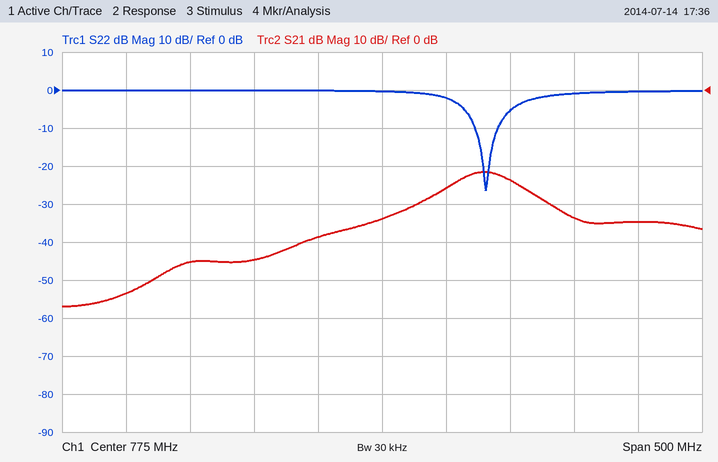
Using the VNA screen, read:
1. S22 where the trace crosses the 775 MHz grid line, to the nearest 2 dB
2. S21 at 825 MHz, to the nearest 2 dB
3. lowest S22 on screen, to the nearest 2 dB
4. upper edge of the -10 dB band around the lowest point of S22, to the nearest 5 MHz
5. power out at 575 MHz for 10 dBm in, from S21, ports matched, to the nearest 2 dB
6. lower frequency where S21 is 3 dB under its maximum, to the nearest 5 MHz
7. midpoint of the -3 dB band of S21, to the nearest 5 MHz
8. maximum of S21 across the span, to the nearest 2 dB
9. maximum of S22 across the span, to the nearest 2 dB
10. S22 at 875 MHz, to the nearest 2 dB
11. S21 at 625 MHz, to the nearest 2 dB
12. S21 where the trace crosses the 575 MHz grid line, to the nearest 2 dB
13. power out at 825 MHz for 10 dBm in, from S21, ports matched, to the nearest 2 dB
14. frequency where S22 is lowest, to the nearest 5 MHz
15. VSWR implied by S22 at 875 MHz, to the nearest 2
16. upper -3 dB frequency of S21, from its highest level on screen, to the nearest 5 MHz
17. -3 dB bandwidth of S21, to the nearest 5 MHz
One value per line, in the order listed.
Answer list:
0 dB
-26 dB
-26 dB
865 MHz
-44 dBm
830 MHz
855 MHz
-22 dB
0 dB
-6 dB
-46 dB
-54 dB
-16 dBm
855 MHz
4
880 MHz
50 MHz
